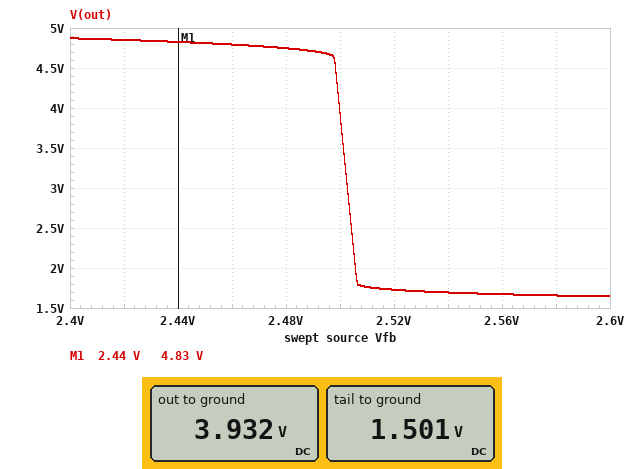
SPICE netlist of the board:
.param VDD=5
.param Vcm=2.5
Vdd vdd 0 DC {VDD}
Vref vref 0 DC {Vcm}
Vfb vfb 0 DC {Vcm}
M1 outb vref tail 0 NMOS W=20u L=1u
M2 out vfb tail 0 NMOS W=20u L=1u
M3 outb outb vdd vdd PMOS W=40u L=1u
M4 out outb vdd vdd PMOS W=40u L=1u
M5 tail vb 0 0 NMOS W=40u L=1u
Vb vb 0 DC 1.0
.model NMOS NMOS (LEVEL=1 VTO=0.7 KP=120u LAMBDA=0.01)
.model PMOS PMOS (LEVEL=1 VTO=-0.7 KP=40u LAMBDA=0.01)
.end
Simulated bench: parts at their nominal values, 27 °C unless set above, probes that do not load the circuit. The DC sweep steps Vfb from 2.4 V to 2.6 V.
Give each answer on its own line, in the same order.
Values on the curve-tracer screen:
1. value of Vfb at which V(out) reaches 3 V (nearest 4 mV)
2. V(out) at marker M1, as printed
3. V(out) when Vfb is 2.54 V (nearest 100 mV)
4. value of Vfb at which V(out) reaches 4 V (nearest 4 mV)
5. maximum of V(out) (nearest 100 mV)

2.504 V
4.83 V
1.7 V
2.500 V
4.9 V
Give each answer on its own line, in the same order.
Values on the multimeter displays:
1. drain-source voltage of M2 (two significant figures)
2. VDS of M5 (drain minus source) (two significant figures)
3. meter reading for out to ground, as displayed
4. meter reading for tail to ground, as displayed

2.4 V
1.5 V
3.932 V
1.501 V
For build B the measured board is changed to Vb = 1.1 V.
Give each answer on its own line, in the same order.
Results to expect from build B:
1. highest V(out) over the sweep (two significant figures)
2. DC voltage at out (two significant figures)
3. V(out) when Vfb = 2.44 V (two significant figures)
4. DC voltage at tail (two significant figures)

4.8 V
3.8 V
4.7 V
1.4 V
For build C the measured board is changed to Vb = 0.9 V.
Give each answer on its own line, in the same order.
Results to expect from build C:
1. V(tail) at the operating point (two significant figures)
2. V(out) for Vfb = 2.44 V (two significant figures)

1.6 V
4.9 V
